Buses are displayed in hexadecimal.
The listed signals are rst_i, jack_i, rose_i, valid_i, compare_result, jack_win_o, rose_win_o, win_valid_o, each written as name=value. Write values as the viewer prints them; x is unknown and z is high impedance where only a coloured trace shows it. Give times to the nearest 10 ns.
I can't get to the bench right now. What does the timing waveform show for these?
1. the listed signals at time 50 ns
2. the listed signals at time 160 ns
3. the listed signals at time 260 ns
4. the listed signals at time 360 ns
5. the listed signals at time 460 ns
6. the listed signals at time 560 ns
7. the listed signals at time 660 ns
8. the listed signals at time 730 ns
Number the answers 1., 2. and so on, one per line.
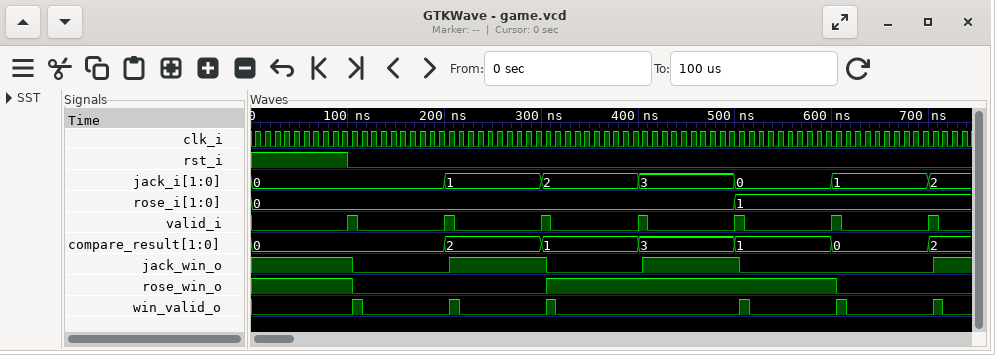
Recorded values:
1. rst_i=1, jack_i=0, rose_i=0, valid_i=0, compare_result=0, jack_win_o=1, rose_win_o=1, win_valid_o=0
2. rst_i=0, jack_i=0, rose_i=0, valid_i=0, compare_result=0, jack_win_o=0, rose_win_o=0, win_valid_o=0
3. rst_i=0, jack_i=1, rose_i=0, valid_i=0, compare_result=2, jack_win_o=1, rose_win_o=0, win_valid_o=0
4. rst_i=0, jack_i=2, rose_i=0, valid_i=0, compare_result=1, jack_win_o=0, rose_win_o=1, win_valid_o=0
5. rst_i=0, jack_i=3, rose_i=0, valid_i=0, compare_result=3, jack_win_o=1, rose_win_o=1, win_valid_o=0
6. rst_i=0, jack_i=0, rose_i=1, valid_i=0, compare_result=1, jack_win_o=0, rose_win_o=1, win_valid_o=0
7. rst_i=0, jack_i=1, rose_i=1, valid_i=0, compare_result=0, jack_win_o=0, rose_win_o=0, win_valid_o=0
8. rst_i=0, jack_i=2, rose_i=1, valid_i=0, compare_result=2, jack_win_o=1, rose_win_o=0, win_valid_o=0
